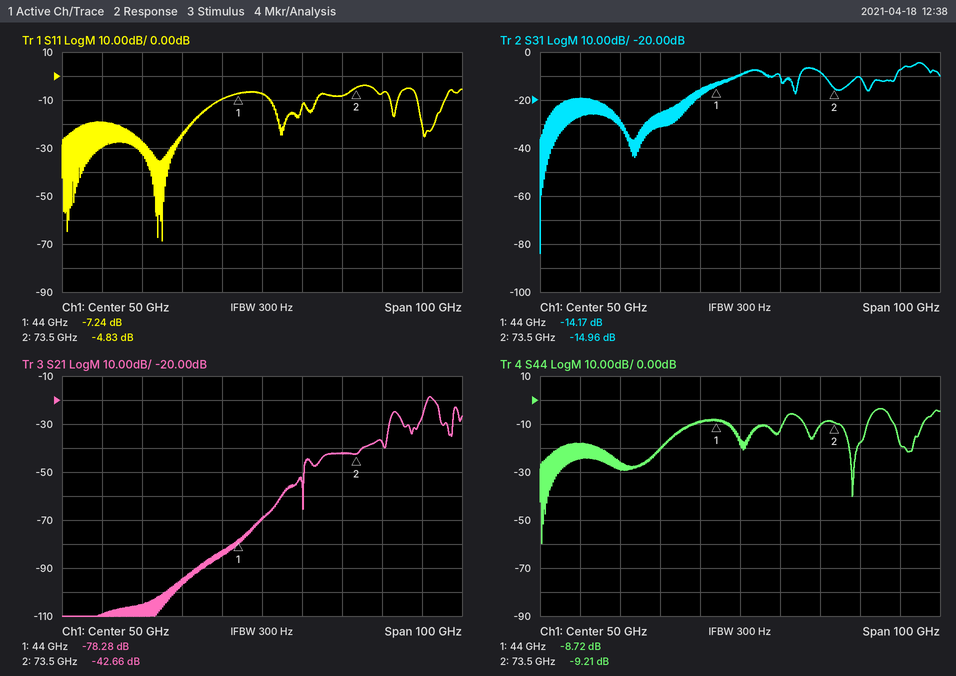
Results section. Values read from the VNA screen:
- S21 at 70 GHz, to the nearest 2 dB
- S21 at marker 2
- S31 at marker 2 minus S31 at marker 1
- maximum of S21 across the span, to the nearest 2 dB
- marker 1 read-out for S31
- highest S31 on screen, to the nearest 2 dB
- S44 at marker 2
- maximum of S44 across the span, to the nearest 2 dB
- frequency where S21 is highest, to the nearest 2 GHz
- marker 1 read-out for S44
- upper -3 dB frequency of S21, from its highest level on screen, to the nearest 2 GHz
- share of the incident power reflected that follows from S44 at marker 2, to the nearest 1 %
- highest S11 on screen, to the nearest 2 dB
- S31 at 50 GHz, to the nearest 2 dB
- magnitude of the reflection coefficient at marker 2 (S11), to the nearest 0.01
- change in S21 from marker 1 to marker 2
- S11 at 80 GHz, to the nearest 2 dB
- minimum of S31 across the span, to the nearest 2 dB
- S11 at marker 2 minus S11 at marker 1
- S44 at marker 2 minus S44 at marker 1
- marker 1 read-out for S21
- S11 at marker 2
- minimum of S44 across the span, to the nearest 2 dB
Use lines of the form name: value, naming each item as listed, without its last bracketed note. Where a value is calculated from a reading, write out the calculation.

S21 at 70 GHz, to the nearest 2 dB: -42 dB
S21 at marker 2: -42.66 dB
S31 at marker 2 minus S31 at marker 1: -14.96 − (-14.17) = -0.79 dB
maximum of S21 across the span, to the nearest 2 dB: -18 dB
marker 1 read-out for S31: -14.17 dB
highest S31 on screen, to the nearest 2 dB: -4 dB
S44 at marker 2: -9.21 dB
maximum of S44 across the span, to the nearest 2 dB: -4 dB
frequency where S21 is highest, to the nearest 2 GHz: 92 GHz
marker 1 read-out for S44: -8.72 dB
upper -3 dB frequency of S21, from its highest level on screen, to the nearest 2 GHz: 94 GHz
share of the incident power reflected that follows from S44 at marker 2, to the nearest 1 %: 10^(-9.21/10) ≈ 12 %
highest S11 on screen, to the nearest 2 dB: -4 dB
S31 at 50 GHz, to the nearest 2 dB: -10 dB
magnitude of the reflection coefficient at marker 2 (S11), to the nearest 0.01: 10^(-4.83/20) ≈ 0.57
change in S21 from marker 1 to marker 2: -42.66 − (-78.28) = 35.62 dB
S11 at 80 GHz, to the nearest 2 dB: -8 dB
minimum of S31 across the span, to the nearest 2 dB: -84 dB
S11 at marker 2 minus S11 at marker 1: -4.83 − (-7.24) = 2.41 dB
S44 at marker 2 minus S44 at marker 1: -9.21 − (-8.72) = -0.49 dB
marker 1 read-out for S21: -78.28 dB
S11 at marker 2: -4.83 dB
minimum of S44 across the span, to the nearest 2 dB: -60 dB
